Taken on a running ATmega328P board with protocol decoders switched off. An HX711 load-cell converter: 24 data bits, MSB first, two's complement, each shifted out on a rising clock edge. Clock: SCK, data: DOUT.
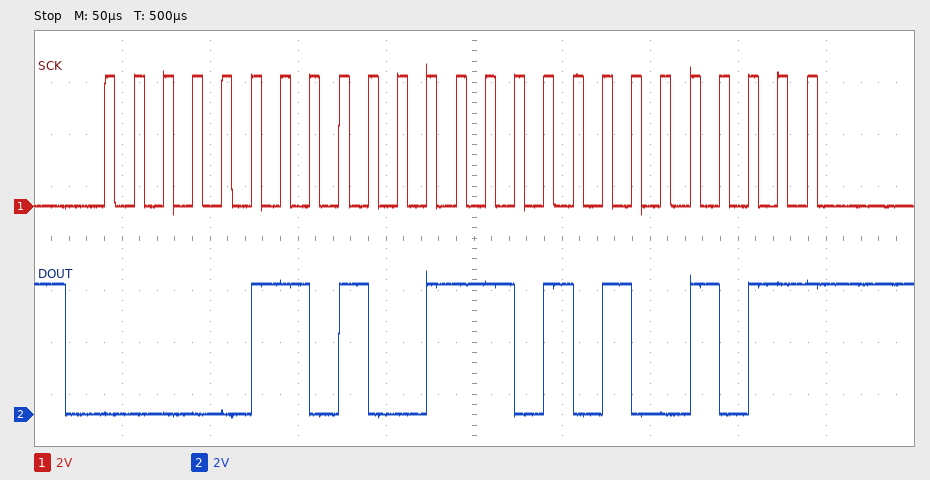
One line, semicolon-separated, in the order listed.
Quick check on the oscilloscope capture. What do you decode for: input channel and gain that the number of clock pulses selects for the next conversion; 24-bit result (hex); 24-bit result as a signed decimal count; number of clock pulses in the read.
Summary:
channel A, gain 128; 0x069D4B; 433483; 25
